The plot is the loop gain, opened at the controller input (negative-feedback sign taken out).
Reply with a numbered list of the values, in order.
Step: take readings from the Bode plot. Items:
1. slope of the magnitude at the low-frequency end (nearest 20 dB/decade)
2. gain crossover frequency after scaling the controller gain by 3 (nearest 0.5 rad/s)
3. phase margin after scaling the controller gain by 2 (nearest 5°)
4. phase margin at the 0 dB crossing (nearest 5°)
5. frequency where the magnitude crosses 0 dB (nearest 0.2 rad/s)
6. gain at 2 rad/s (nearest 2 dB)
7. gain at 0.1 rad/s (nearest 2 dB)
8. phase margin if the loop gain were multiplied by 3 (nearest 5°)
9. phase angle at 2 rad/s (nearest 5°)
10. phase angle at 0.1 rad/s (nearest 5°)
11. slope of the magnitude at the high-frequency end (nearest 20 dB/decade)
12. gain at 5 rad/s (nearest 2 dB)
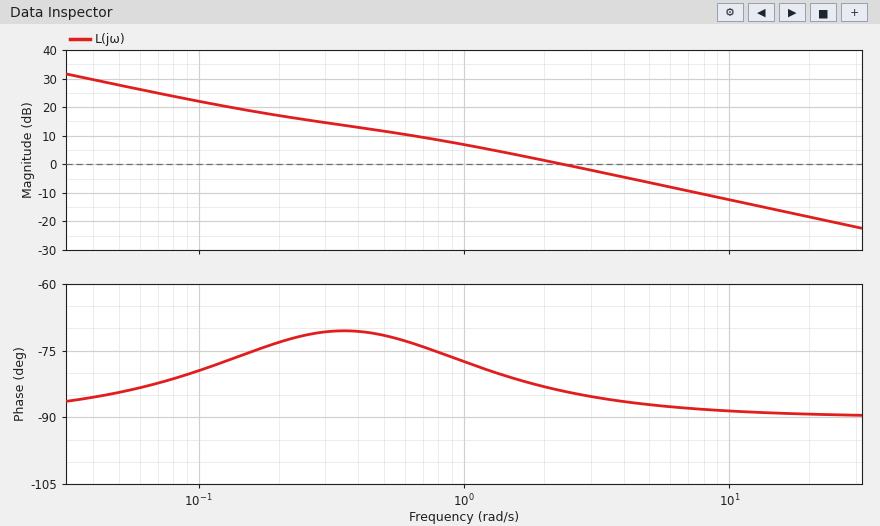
1. -20 dB/decade
2. 7.0 rad/s
3. 95°
4. 95°
5. 2.4 rad/s
6. 2 dB
7. 22 dB
8. 90°
9. -85°
10. -80°
11. -20 dB/decade
12. -6 dB
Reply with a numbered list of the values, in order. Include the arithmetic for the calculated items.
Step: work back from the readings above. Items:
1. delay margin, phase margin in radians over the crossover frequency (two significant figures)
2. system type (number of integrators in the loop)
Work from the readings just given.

1. 95 × π / 180 / 2.4 = 0.69 s
2. 1
